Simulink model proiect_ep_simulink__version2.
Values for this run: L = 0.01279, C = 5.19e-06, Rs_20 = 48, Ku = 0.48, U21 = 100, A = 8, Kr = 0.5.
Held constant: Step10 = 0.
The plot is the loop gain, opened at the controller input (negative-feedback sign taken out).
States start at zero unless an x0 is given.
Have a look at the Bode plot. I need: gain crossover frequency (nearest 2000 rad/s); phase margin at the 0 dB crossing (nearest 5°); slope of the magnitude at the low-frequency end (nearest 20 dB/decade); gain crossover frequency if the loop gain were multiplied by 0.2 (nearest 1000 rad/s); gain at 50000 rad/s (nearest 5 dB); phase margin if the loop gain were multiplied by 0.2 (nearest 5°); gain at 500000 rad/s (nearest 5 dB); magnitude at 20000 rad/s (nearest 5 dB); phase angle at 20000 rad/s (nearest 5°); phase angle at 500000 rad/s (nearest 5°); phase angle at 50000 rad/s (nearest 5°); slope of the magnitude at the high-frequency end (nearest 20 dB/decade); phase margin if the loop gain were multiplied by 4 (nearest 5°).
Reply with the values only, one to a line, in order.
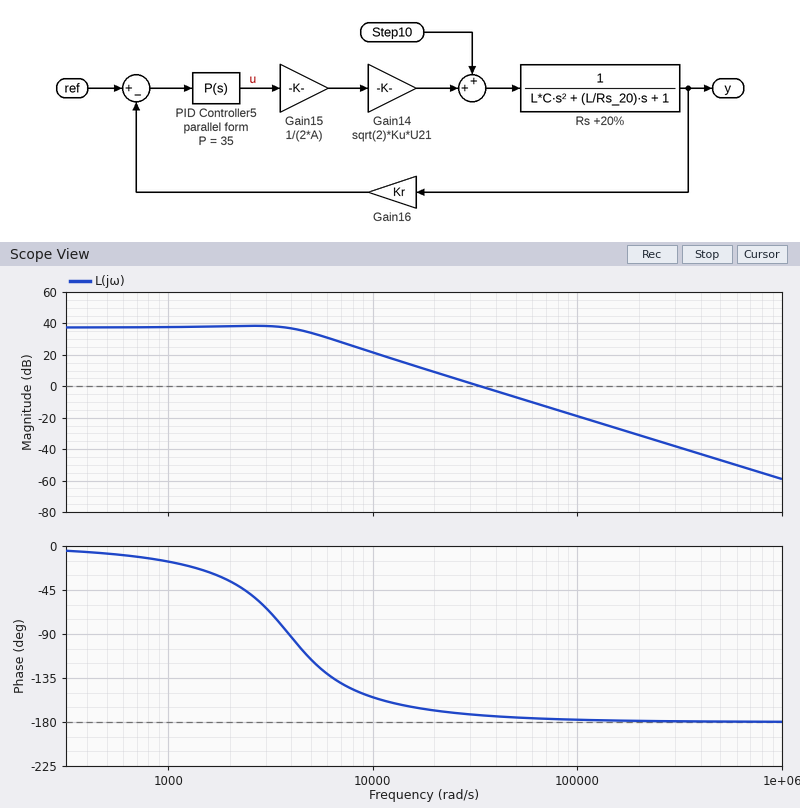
34000 rad/s
5°
0 dB/decade
15000 rad/s
-5 dB
15°
-45 dB
10 dB
-170°
-180°
-175°
-40 dB/decade
5°
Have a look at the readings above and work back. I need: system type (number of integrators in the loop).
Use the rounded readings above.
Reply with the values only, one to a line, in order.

0
